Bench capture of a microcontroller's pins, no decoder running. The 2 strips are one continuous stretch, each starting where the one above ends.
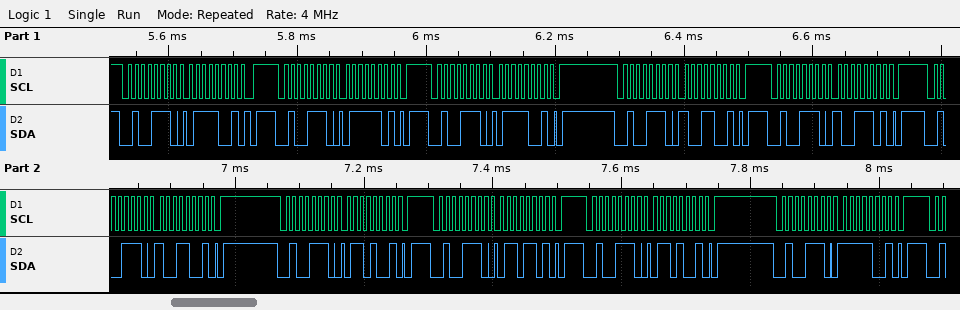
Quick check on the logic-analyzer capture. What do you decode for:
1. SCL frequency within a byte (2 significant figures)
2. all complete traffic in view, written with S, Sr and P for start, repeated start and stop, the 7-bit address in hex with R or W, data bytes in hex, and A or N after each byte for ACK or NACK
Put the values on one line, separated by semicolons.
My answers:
100 kHz; S 27W A 79 A P S 27W A 7D A P S 27W A 79 A P S 27W A 99 A P S 27W A 9D A P S 27W A 99 A P S 27W A 69 A P S 27W A 6D A P S 27W A 69 A P S 27W A F9 A P
